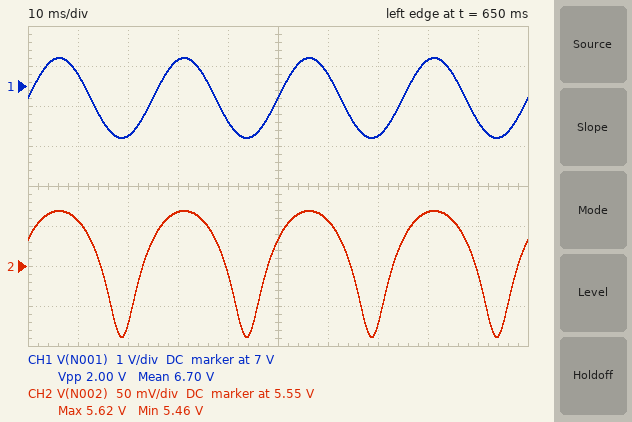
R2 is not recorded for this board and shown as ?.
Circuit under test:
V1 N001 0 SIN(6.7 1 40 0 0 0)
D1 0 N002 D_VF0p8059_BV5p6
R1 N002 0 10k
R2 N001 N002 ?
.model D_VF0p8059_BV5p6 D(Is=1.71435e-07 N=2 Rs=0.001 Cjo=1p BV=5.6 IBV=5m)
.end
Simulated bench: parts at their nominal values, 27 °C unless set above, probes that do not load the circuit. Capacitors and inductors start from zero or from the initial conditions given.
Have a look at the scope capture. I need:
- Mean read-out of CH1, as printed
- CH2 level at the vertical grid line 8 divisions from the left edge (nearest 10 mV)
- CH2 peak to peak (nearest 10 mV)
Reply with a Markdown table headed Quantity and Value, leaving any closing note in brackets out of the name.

| Quantity | Value |
|---|---|
| Mean read-out of CH1, as printed | 6.70 V |
| CH2 level at the vertical grid line 8 divisions from the left edge | 5.62 V |
| CH2 peak to peak | 160 mV |
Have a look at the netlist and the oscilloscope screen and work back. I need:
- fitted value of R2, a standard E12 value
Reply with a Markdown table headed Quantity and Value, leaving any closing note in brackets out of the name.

| Quantity | Value |
|---|---|
| fitted value of R2, a standard E12 value | 270 Ω |
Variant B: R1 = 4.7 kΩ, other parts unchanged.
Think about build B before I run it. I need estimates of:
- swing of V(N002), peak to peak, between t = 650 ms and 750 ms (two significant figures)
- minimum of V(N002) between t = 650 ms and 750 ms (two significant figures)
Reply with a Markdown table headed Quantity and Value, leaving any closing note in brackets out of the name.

| Quantity | Value |
|---|---|
| swing of V(N002), peak to peak, between t = 650 ms and 750 ms | 240 mV |
| minimum of V(N002) between t = 650 ms and 750 ms | 5.4 V |
